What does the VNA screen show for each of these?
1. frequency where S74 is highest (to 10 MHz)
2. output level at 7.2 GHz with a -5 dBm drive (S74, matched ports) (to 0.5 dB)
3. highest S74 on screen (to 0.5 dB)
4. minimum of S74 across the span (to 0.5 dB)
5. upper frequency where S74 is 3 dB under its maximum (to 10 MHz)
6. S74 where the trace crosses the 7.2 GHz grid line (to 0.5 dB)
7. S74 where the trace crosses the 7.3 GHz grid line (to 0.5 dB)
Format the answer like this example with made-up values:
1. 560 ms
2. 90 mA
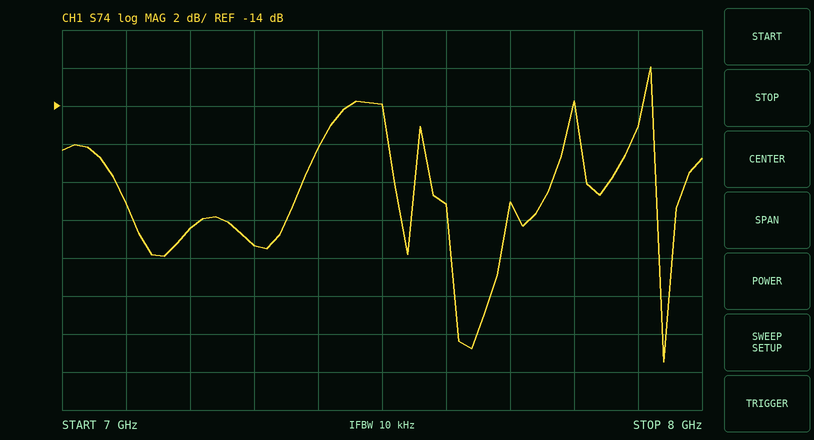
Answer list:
1. 7.92 GHz
2. -25.5 dBm
3. -12.0 dB
4. -27.5 dB
5. 7.92 GHz
6. -20.5 dB
7. -21.5 dB
